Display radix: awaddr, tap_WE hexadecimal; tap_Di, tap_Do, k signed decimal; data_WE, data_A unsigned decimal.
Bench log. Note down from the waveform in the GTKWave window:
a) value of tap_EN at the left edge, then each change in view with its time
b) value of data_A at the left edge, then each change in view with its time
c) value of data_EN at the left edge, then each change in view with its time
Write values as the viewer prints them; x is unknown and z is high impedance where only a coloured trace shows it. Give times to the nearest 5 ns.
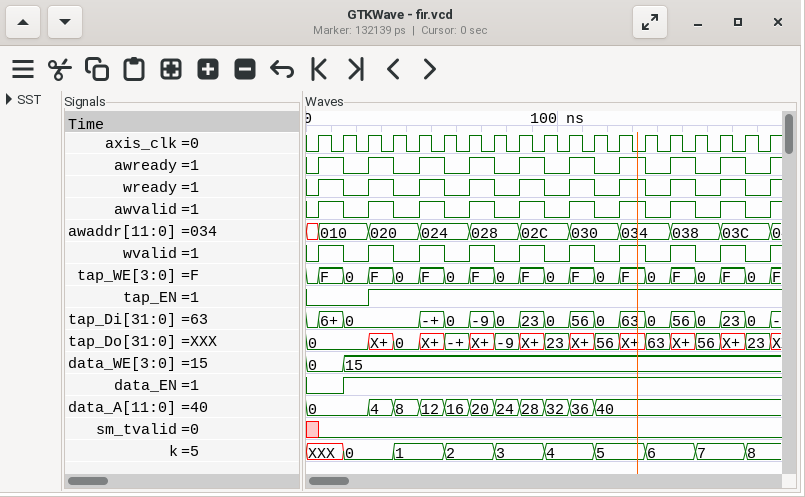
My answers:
0, 1 at 25 ns
0, 4 at 25 ns, 8 at 35 ns, 12 at 45 ns, 16 at 55 ns, 20 at 65 ns, 24 at 75 ns, 28 at 85 ns, 32 at 95 ns, 36 at 105 ns, 40 at 115 ns
0, 1 at 15 ns
